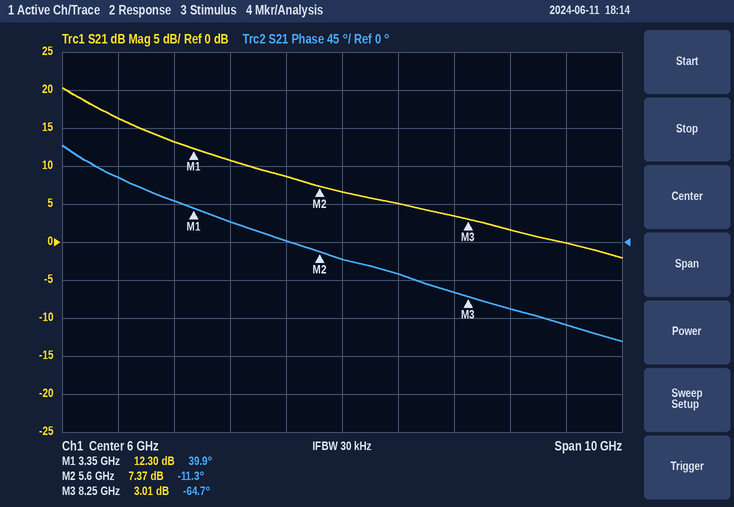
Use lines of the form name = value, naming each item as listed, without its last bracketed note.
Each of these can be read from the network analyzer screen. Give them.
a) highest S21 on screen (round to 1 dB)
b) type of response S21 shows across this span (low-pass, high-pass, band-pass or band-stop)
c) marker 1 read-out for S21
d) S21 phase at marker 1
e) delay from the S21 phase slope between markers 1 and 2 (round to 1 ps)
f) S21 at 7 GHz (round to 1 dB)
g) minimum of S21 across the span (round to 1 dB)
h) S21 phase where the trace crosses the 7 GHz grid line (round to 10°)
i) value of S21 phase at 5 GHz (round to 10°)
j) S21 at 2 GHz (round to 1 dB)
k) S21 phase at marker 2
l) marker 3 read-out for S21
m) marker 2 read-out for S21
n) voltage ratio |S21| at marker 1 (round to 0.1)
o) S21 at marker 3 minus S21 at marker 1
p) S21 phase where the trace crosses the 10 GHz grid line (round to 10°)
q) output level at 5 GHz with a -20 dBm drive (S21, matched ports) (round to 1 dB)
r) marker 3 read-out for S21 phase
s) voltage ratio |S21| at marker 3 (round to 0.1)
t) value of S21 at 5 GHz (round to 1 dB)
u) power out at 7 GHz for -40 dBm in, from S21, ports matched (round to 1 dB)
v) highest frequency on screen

highest S21 on screen = 20 dB
type of response S21 shows across this span = low-pass
marker 1 read-out for S21 = 12.30 dB
S21 phase at marker 1 = 39.9°
delay from the S21 phase slope between markers 1 and 2 = 63 ps
S21 at 7 GHz = 5 dB
minimum of S21 across the span = -2 dB
S21 phase where the trace crosses the 7 GHz grid line = -40°
value of S21 phase at 5 GHz = 0°
S21 at 2 GHz = 16 dB
S21 phase at marker 2 = -11.3°
marker 3 read-out for S21 = 3.01 dB
marker 2 read-out for S21 = 7.37 dB
voltage ratio |S21| at marker 1 = 4.1
S21 at marker 3 minus S21 at marker 1 = -9.29 dB
S21 phase where the trace crosses the 10 GHz grid line = -100°
output level at 5 GHz with a -20 dBm drive (S21, matched ports) = -11 dBm
marker 3 read-out for S21 phase = -64.7°
voltage ratio |S21| at marker 3 = 1.4
value of S21 at 5 GHz = 9 dB
power out at 7 GHz for -40 dBm in, from S21, ports matched = -35 dBm
highest frequency on screen = 11 GHz
